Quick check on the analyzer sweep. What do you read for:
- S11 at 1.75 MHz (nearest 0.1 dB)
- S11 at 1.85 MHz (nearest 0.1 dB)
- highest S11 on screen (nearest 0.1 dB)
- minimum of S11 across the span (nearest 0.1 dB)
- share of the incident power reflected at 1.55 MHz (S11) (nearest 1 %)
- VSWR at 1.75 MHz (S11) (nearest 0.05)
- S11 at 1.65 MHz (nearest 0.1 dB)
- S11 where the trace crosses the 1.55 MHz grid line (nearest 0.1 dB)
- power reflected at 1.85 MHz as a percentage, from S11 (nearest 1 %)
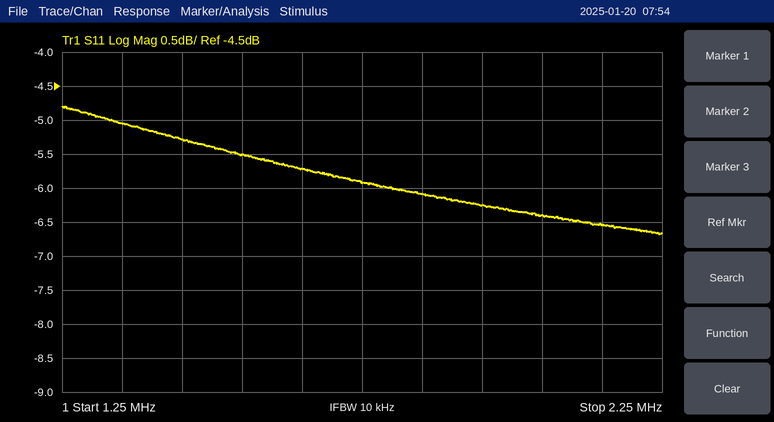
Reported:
-5.9 dB
-6.1 dB
-4.8 dB
-6.7 dB
28 %
3.05
-5.7 dB
-5.5 dB
25 %
